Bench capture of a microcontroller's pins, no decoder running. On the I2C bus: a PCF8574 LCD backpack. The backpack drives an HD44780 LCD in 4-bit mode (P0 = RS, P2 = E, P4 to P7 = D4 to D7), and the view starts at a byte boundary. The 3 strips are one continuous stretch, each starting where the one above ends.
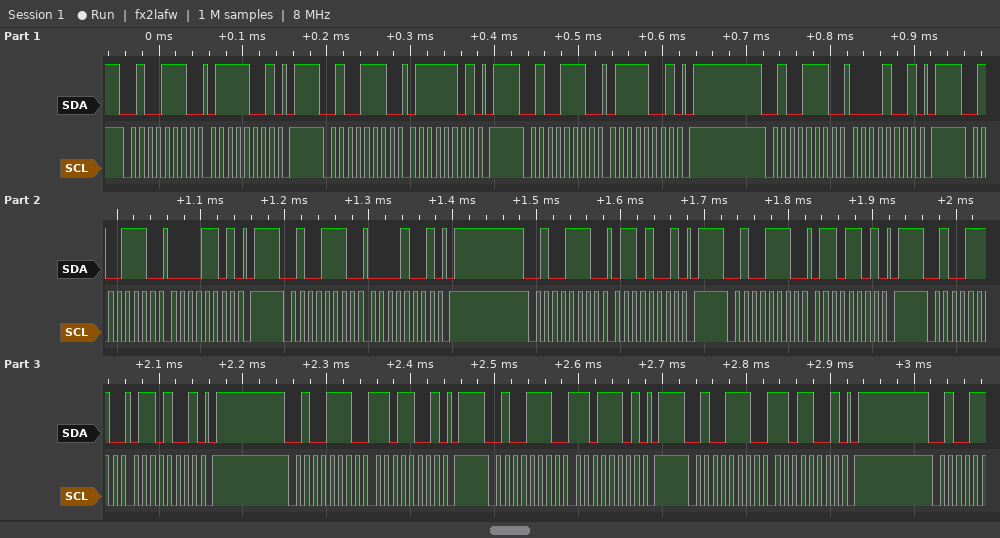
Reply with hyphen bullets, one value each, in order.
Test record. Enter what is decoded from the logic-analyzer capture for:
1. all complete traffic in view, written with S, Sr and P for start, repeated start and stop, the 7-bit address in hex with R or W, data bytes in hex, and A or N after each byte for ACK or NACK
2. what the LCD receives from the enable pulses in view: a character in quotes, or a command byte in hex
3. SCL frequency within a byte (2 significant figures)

- S 27W A 79 A P S 27W A 7D A P S 27W A 79 A P S 27W A 09 A P S 27W A 0D A P S 27W A 09 A P S 27W A 69 A P S 27W A 6D A P S 27W A 69 A P S 27W A D9 A P S 27W A DD A P S 27W A D9 A P
- 'p' 'm'
- 100 kHz
